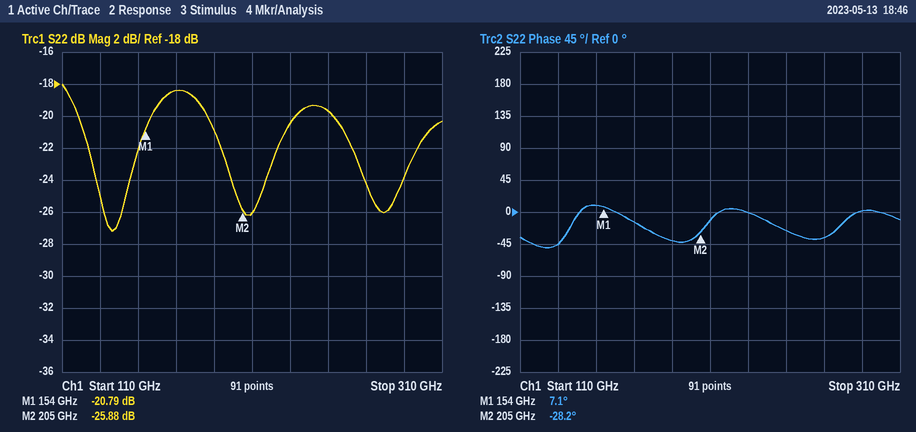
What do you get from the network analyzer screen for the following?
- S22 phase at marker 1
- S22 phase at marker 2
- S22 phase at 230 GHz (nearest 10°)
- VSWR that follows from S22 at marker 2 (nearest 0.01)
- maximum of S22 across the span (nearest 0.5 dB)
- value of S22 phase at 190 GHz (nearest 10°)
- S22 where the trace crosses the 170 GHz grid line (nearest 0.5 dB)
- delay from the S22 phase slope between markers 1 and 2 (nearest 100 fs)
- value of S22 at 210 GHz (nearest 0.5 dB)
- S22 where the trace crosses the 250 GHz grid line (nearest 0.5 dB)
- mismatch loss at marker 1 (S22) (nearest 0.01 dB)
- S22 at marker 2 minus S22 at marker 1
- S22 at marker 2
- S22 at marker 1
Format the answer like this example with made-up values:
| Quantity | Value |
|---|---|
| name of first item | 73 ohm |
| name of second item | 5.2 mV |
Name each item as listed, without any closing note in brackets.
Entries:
| Quantity | Value |
|---|---|
| S22 phase at marker 1 | 7.1° |
| S22 phase at marker 2 | -28.2° |
| S22 phase at 230 GHz | 0° |
| VSWR that follows from S22 at marker 2 | 1.11 |
| maximum of S22 across the span | -18.0 dB |
| value of S22 phase at 190 GHz | -40° |
| S22 where the trace crosses the 170 GHz grid line | -18.5 dB |
| delay from the S22 phase slope between markers 1 and 2 | 1.9 ps |
| value of S22 at 210 GHz | -26.0 dB |
| S22 where the trace crosses the 250 GHz grid line | -19.5 dB |
| mismatch loss at marker 1 (S22) | 0.04 dB |
| S22 at marker 2 minus S22 at marker 1 | -5.09 dB |
| S22 at marker 2 | -25.88 dB |
| S22 at marker 1 | -20.79 dB |
